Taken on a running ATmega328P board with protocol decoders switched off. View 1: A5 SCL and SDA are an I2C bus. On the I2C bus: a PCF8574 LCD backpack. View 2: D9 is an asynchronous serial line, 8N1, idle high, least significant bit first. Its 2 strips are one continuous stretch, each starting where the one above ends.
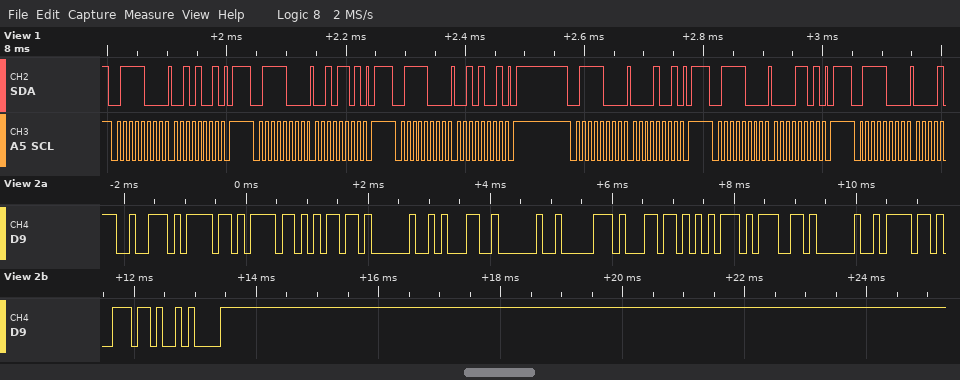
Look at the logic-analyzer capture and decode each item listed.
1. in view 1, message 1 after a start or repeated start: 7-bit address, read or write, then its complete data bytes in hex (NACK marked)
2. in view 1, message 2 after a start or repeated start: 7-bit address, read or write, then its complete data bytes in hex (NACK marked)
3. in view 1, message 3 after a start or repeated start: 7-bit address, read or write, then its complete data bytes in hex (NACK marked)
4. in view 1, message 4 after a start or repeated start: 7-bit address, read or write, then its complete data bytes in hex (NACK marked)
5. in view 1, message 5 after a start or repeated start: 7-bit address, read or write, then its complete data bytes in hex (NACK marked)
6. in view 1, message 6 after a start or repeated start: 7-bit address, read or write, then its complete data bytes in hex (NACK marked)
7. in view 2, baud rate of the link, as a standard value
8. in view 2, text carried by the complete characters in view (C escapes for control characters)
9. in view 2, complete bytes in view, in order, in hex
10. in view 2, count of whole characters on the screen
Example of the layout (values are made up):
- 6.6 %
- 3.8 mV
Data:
- 0x3C write: 29
- 0x3C write: 2D
- 0x3C write: 29
- 0x3C write: 09
- 0x3C write: 0D
- 0x3C write
- 9600 baud
- "room 1 plug on\n"
- 72 6F 6F 6D 20 31 20 70 6C 75 67 20 6F 6E 0A
- 15
